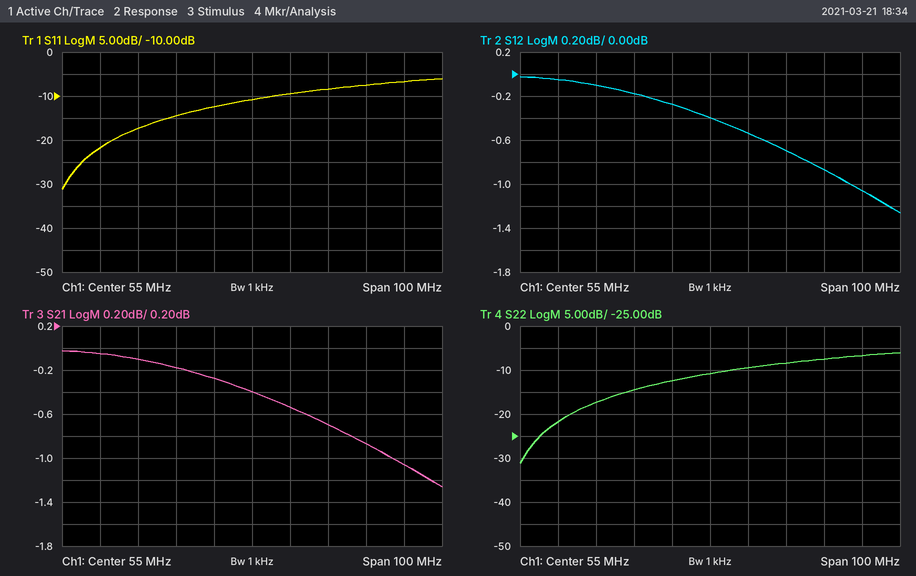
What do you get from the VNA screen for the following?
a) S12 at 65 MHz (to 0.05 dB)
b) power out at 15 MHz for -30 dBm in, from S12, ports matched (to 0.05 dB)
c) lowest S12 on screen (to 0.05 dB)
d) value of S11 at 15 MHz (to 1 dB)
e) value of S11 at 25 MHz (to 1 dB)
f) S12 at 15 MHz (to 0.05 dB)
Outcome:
-0.55 dB
-30.05 dBm
-1.25 dB
-22 dB
-17 dB
-0.05 dB
